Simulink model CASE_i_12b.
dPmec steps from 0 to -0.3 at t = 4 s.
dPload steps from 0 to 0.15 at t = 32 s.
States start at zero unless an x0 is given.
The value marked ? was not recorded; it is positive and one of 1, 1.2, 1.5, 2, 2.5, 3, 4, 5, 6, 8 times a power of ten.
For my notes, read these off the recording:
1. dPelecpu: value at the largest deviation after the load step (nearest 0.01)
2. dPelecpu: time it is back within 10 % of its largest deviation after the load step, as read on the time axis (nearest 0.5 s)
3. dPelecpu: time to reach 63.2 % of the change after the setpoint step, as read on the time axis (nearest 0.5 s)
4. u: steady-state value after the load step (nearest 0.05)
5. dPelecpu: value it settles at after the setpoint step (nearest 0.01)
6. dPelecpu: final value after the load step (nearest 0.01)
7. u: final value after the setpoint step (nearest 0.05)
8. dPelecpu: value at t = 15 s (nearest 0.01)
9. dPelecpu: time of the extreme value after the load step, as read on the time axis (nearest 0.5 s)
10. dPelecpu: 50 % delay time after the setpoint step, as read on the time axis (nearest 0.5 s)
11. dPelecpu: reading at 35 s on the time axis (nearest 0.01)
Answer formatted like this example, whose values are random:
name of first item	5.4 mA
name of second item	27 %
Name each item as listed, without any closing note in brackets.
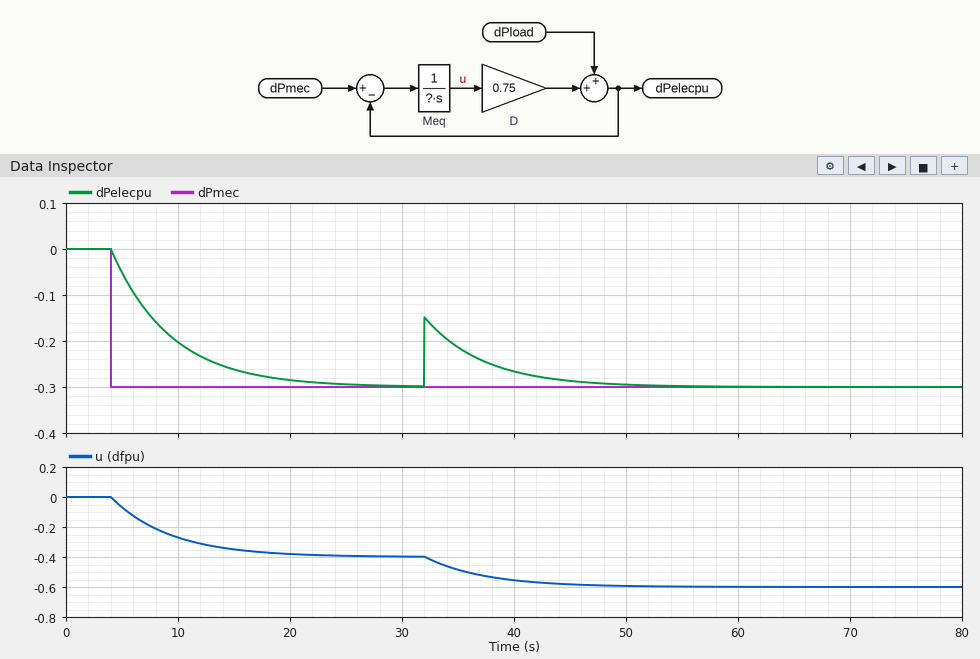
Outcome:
dPelecpu: value at the largest deviation after the load step	-0.15
dPelecpu: time it is back within 10 % of its largest deviation after the load step, as read on the time axis	44.5 s
dPelecpu: time to reach 63.2 % of the change after the setpoint step, as read on the time axis	9.5 s
u: steady-state value after the load step	-0.60
dPelecpu: value it settles at after the setpoint step	-0.30
dPelecpu: final value after the load step	-0.30
u: final value after the setpoint step	-0.40
dPelecpu: value at t = 15 s	-0.26
dPelecpu: time of the extreme value after the load step, as read on the time axis	32.0 s
dPelecpu: 50 % delay time after the setpoint step, as read on the time axis	7.5 s
dPelecpu: reading at 35 s on the time axis	-0.21
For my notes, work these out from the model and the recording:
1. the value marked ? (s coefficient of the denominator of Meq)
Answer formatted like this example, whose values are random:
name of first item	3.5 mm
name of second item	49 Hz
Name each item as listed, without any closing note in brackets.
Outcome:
the value marked ?	4
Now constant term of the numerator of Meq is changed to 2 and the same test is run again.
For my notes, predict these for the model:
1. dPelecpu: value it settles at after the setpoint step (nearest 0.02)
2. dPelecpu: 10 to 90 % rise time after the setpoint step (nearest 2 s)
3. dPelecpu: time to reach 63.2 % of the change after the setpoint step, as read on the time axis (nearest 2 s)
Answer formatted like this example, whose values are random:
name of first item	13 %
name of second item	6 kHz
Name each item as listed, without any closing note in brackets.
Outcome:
dPelecpu: value it settles at after the setpoint step	-0.30
dPelecpu: 10 to 90 % rise time after the setpoint step	6 s
dPelecpu: time to reach 63.2 % of the change after the setpoint step, as read on the time axis	6 s
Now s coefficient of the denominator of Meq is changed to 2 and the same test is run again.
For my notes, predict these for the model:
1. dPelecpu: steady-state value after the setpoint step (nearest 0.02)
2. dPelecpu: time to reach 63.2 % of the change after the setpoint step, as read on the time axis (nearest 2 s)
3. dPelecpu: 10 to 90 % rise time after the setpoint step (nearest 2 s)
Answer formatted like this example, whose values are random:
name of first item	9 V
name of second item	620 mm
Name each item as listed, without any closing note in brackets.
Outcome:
dPelecpu: steady-state value after the setpoint step	-0.30
dPelecpu: time to reach 63.2 % of the change after the setpoint step, as read on the time axis	6 s
dPelecpu: 10 to 90 % rise time after the setpoint step	6 s
